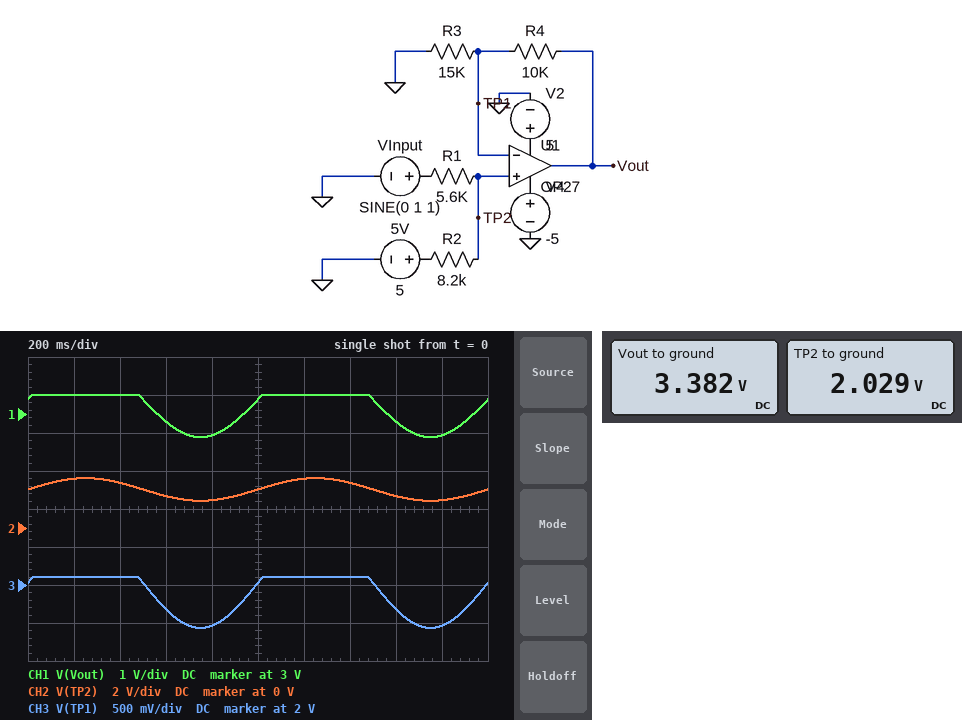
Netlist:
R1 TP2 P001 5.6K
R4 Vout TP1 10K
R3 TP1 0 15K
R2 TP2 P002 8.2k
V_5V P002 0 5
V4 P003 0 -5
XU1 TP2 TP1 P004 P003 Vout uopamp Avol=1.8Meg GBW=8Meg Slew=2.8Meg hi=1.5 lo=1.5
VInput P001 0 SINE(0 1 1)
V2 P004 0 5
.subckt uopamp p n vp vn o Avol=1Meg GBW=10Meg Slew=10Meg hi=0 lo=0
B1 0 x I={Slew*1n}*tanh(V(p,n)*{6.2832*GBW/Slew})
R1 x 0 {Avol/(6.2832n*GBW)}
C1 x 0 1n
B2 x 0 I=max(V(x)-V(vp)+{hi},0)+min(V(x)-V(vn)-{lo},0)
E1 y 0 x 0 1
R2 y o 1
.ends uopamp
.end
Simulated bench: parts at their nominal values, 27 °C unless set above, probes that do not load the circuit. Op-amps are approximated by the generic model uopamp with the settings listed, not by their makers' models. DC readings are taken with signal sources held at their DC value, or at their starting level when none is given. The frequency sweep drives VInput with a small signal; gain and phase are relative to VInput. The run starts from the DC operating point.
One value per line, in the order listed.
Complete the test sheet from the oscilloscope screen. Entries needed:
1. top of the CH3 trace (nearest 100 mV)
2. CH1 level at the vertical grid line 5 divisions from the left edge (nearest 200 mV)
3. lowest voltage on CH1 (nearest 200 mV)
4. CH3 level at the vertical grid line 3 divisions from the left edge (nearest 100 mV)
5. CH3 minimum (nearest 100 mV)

2.1 V
3.4 V
2.4 V
1.7 V
1.4 V
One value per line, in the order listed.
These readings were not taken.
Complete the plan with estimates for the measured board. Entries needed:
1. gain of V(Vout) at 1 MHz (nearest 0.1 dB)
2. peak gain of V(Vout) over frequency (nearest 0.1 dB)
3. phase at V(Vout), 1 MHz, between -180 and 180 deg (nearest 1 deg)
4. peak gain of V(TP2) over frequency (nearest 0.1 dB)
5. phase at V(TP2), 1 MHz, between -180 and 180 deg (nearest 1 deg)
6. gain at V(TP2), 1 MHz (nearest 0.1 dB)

-0.3 dB
-0.1 dB
-12 deg
-4.5 dB
0 deg
-4.5 dB
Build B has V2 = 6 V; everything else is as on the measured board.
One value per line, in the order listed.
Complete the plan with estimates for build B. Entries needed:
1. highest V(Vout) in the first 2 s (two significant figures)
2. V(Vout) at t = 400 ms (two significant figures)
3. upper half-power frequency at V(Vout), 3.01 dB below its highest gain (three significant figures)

4.4 V
4.0 V
4.80 MHz
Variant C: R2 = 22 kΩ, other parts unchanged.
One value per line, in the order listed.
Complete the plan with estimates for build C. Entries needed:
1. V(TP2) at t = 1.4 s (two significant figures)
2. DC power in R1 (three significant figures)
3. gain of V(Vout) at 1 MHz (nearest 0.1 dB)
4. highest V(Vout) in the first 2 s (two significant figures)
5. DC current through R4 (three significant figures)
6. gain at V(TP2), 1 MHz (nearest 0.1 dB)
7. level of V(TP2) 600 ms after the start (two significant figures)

1.5 V
184 µW
2.3 dB
3.0 V
67.6 µA
-2.0 dB
550 mV
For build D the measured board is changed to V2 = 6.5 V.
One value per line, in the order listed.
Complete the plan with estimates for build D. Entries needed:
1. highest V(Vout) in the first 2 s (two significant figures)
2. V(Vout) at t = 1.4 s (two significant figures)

4.4 V
4.0 V
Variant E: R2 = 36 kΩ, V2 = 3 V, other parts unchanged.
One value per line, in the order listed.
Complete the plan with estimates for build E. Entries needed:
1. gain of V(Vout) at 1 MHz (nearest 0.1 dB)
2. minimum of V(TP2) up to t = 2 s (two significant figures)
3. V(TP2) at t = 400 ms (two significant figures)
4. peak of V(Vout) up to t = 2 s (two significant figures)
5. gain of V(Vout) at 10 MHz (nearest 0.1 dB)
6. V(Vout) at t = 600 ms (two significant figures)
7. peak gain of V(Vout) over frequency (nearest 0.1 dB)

3.0 dB
-190 mV
1.2 V
1.5 V
-4.1 dB
270 mV
3.2 dB
